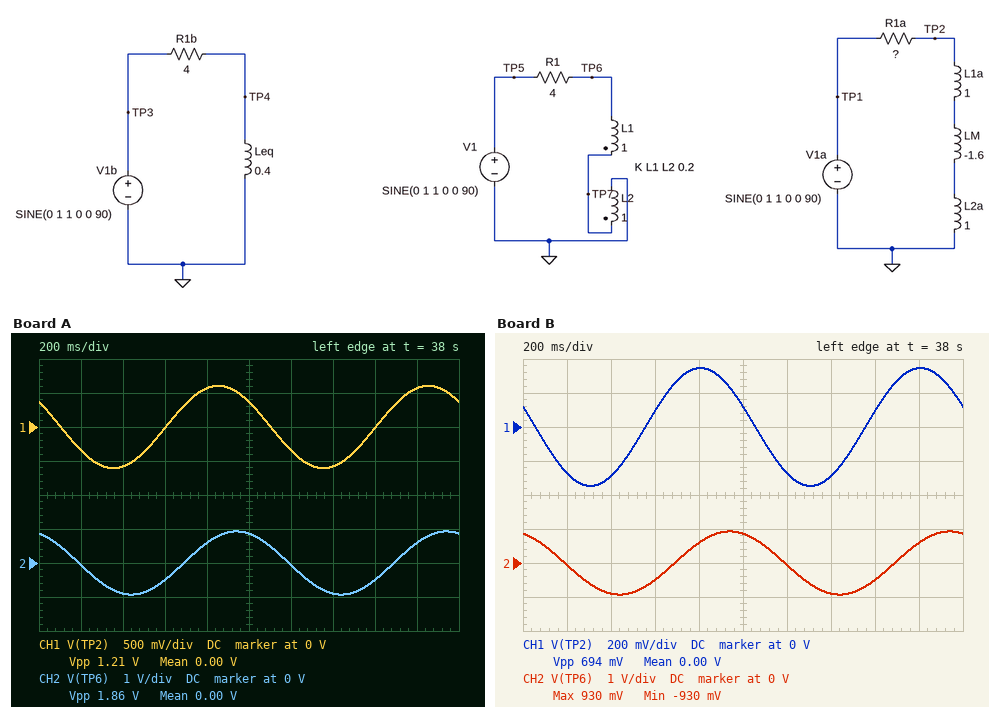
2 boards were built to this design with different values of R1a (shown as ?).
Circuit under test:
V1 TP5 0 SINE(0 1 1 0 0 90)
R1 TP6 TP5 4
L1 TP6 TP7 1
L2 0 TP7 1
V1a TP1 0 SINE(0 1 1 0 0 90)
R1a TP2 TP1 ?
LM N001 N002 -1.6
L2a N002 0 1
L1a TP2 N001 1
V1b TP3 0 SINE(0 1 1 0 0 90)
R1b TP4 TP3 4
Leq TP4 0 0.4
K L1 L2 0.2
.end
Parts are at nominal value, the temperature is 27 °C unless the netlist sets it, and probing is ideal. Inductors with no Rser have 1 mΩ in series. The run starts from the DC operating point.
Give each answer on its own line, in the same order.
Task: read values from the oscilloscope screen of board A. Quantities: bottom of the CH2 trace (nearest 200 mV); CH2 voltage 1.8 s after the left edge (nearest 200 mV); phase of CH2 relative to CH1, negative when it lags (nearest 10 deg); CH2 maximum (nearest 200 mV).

-1.0 V
600 mV
-30 deg
1.0 V
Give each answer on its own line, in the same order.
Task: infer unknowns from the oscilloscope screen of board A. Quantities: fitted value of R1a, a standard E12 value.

3.3 Ω
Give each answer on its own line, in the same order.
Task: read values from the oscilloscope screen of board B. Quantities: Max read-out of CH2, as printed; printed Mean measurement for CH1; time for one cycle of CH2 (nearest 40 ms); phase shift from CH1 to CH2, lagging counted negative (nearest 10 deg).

930 mV
0.00 V
1.00 s
-50 deg
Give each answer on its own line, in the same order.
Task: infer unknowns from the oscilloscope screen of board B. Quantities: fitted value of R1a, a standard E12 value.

6.8 Ω
